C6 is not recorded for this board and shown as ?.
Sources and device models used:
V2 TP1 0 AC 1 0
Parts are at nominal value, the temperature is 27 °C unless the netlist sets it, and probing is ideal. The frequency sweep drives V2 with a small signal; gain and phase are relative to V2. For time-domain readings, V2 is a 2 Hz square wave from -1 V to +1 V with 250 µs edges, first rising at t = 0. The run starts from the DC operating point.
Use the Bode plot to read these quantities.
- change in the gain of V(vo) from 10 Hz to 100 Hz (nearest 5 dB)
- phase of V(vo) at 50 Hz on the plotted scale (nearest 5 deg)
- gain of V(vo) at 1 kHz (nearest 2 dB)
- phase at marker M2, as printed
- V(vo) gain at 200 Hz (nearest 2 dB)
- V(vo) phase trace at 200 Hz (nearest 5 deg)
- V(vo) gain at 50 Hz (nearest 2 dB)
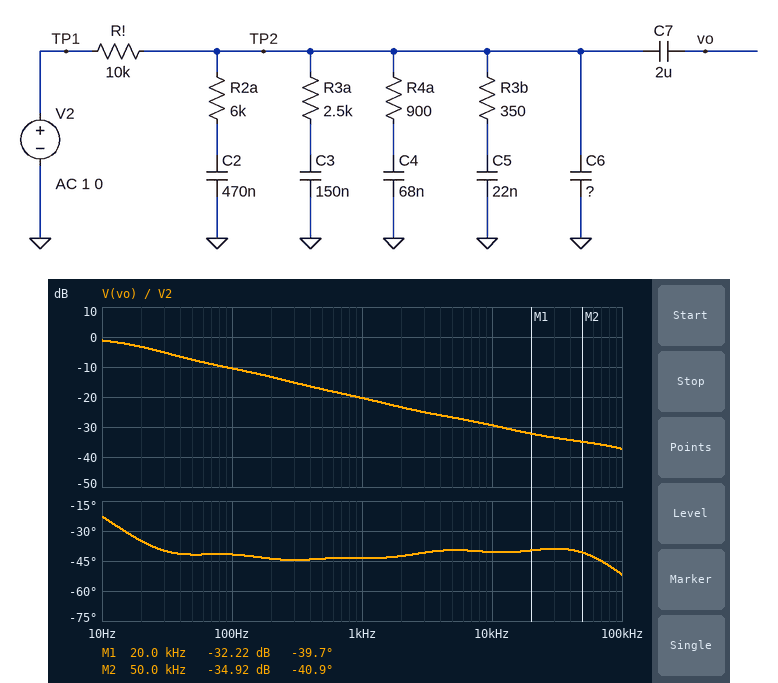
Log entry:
-10 dB
-40 deg
-20 dB
-40.9 deg
-14 dB
-45 deg
-8 dB
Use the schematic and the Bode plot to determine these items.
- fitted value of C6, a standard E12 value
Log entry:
8.2 nF
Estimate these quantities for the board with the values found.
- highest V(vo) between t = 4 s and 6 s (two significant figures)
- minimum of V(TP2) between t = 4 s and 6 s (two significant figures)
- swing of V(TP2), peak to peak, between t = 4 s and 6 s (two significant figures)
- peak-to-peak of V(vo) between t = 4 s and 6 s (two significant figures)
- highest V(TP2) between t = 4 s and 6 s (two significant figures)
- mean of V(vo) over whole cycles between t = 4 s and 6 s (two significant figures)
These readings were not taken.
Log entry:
2.0 V
-1.0 V
2.0 V
2.0 V
1.0 V
1.0 V
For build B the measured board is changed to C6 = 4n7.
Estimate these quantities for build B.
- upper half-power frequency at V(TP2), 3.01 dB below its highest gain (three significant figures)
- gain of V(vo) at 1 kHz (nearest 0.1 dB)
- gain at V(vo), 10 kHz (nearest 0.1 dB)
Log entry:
18.8 Hz
-20.2 dB
-29.0 dB
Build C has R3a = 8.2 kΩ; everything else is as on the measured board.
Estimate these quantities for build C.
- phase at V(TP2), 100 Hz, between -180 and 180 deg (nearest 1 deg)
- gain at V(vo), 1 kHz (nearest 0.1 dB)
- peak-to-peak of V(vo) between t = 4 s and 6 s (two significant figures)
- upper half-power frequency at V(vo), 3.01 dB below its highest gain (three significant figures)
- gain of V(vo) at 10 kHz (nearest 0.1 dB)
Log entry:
-35 deg
-18.0 dB
2.0 V
18.4 Hz
-28.8 dB
